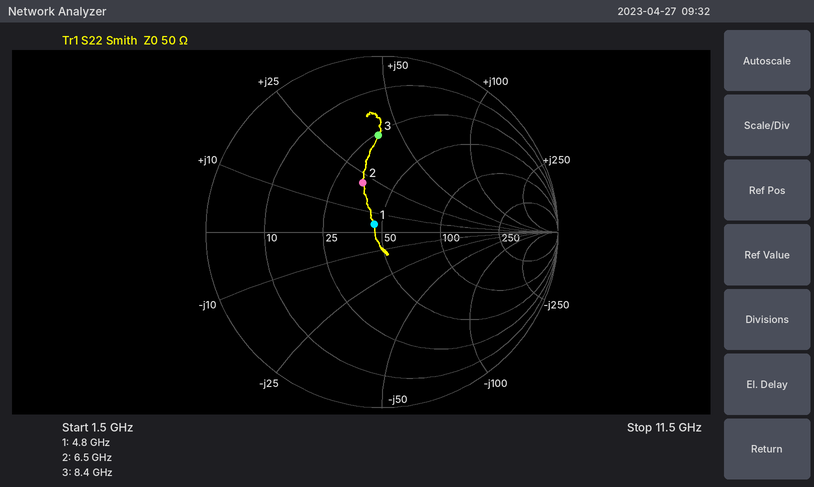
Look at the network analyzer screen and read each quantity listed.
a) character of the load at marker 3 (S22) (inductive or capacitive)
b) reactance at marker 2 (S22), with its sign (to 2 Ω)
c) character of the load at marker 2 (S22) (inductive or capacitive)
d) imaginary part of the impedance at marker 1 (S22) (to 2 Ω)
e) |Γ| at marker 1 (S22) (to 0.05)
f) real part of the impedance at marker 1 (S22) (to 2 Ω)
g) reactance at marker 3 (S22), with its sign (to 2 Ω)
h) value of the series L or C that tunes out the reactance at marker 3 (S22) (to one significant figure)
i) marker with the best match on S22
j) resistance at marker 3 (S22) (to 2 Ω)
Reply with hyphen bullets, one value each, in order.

- inductive
- +22 Ω
- inductive
- +4 Ω
- 0.05
- 46 Ω
- +40 Ω
- 500 fF
- marker 1
- 26 Ω
